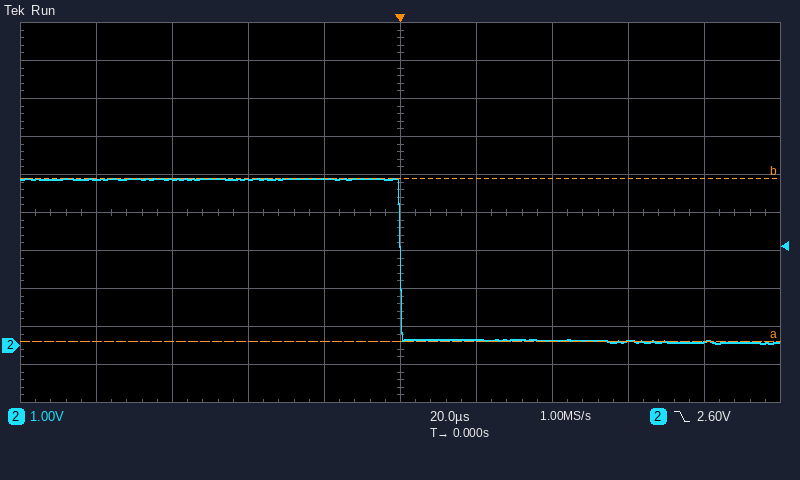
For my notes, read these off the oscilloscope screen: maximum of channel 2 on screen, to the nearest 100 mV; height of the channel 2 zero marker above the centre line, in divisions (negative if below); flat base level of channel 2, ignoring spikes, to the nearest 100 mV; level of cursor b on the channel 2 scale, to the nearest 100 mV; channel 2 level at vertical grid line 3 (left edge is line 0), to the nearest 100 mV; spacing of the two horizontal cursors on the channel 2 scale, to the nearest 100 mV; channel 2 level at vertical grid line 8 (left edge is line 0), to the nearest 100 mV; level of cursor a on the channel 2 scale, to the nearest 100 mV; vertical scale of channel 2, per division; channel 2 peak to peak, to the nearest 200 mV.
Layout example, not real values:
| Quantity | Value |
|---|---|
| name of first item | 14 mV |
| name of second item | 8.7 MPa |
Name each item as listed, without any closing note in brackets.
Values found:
| Quantity | Value |
|---|---|
| maximum of channel 2 on screen, to the nearest 100 mV | 4.4 V |
| height of the channel 2 zero marker above the centre line, in divisions | -3.5 div |
| flat base level of channel 2, ignoring spikes, to the nearest 100 mV | 100 mV |
| level of cursor b on the channel 2 scale, to the nearest 100 mV | 4.4 V |
| channel 2 level at vertical grid line 3 (left edge is line 0), to the nearest 100 mV | 4.4 V |
| spacing of the two horizontal cursors on the channel 2 scale, to the nearest 100 mV | 4.3 V |
| channel 2 level at vertical grid line 8 (left edge is line 0), to the nearest 100 mV | 100 mV |
| level of cursor a on the channel 2 scale, to the nearest 100 mV | 100 mV |
| vertical scale of channel 2, per division | 1 V |
| channel 2 peak to peak, to the nearest 200 mV | 4.4 V |
